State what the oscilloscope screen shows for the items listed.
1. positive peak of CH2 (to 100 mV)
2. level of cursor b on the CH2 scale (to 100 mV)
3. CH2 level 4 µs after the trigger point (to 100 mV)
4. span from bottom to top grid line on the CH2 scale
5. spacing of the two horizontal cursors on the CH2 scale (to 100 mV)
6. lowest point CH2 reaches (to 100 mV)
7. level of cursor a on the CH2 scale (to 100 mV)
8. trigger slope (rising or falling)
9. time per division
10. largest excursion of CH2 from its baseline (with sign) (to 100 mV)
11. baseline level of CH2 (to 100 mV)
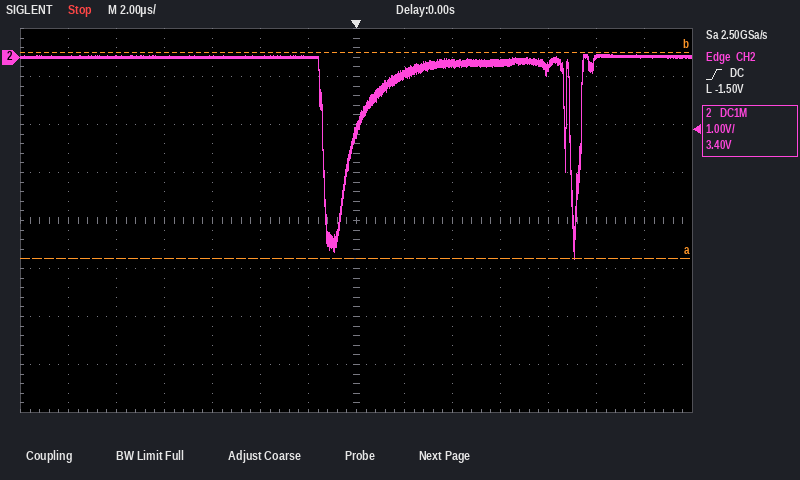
100 mV
100 mV
-100 mV
8 V
4.3 V
-4.2 V
-4.2 V
rising
2 µs
-4.2 V
0.0 V
